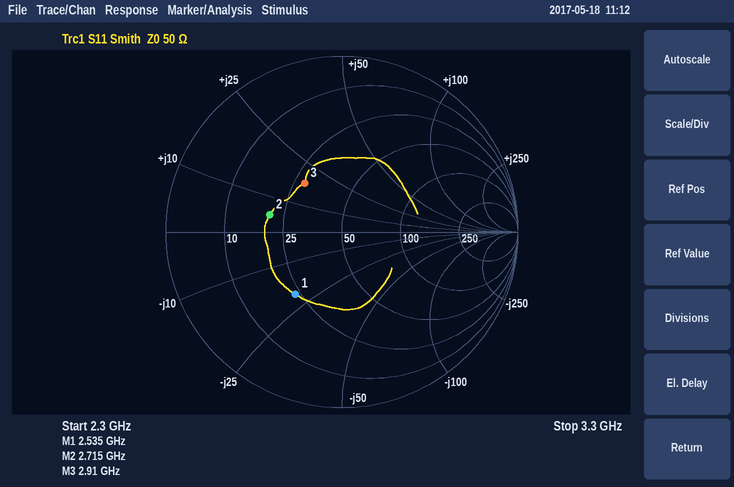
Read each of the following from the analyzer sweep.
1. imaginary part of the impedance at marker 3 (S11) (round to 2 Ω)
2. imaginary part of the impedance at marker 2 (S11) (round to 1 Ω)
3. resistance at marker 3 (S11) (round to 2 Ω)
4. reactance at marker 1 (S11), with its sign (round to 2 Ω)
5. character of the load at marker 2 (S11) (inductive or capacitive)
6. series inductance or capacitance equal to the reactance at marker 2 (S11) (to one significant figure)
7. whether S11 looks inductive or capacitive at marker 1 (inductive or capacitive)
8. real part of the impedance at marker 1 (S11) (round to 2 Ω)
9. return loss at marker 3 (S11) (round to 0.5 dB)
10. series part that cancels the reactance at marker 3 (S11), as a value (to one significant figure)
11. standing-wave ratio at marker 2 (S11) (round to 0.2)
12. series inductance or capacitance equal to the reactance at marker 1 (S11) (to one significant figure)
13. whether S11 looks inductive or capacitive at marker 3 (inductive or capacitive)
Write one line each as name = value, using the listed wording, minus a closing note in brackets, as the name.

imaginary part of the impedance at marker 3 (S11) = +18 Ω
imaginary part of the impedance at marker 2 (S11) = +5 Ω
resistance at marker 3 (S11) = 28 Ω
reactance at marker 1 (S11), with its sign = -20 Ω
character of the load at marker 2 (S11) = inductive
series inductance or capacitance equal to the reactance at marker 2 (S11) = 300 pH
whether S11 looks inductive or capacitive at marker 1 = capacitive
real part of the impedance at marker 1 (S11) = 24 Ω
return loss at marker 3 (S11) = 9.0 dB
series part that cancels the reactance at marker 3 (S11), as a value = 3 pF
standing-wave ratio at marker 2 (S11) = 2.4
series inductance or capacitance equal to the reactance at marker 1 (S11) = 3 pF
whether S11 looks inductive or capacitive at marker 3 = inductive
